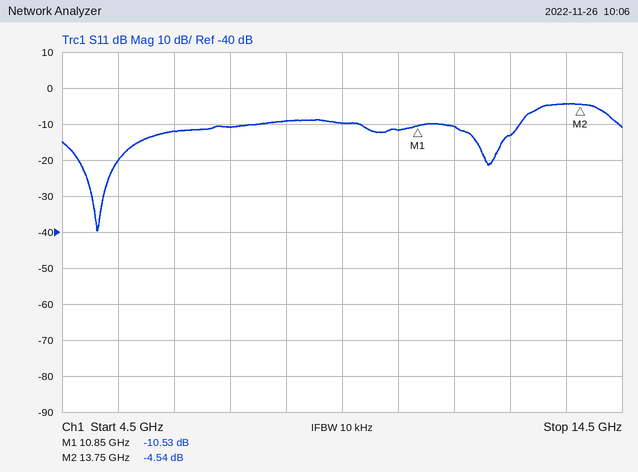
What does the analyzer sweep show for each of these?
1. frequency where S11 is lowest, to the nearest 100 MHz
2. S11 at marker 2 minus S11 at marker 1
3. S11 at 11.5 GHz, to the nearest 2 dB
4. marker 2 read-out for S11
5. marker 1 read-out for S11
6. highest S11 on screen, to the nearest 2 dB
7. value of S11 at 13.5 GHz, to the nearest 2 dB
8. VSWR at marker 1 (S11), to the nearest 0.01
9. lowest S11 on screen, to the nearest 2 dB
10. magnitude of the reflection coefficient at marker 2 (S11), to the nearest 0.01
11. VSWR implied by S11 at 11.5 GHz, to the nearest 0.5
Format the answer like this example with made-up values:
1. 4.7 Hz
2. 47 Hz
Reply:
1. 5.1 GHz
2. 5.99 dB
3. -10 dB
4. -4.54 dB
5. -10.53 dB
6. -4 dB
7. -4 dB
8. 1.85
9. -40 dB
10. 0.59
11. 2.0
